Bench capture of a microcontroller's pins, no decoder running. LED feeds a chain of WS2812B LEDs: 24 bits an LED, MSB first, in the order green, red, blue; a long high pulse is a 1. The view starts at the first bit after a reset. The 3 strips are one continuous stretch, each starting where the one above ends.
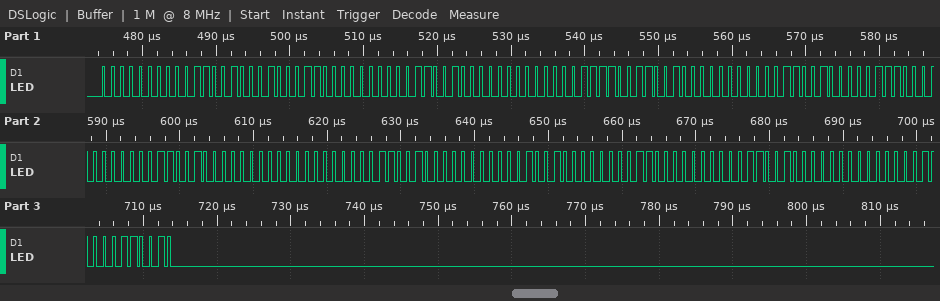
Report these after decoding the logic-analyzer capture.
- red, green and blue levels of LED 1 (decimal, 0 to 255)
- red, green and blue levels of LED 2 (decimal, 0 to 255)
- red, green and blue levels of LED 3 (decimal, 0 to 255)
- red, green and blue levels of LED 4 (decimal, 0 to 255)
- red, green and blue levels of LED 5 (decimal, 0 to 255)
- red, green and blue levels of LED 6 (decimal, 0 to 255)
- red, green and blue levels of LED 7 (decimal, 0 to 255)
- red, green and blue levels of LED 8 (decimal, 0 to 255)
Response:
50, 0, 35
50, 0, 0
50, 15, 0
14, 50, 0
0, 50, 0
0, 50, 36
0, 3, 50
4, 0, 50
